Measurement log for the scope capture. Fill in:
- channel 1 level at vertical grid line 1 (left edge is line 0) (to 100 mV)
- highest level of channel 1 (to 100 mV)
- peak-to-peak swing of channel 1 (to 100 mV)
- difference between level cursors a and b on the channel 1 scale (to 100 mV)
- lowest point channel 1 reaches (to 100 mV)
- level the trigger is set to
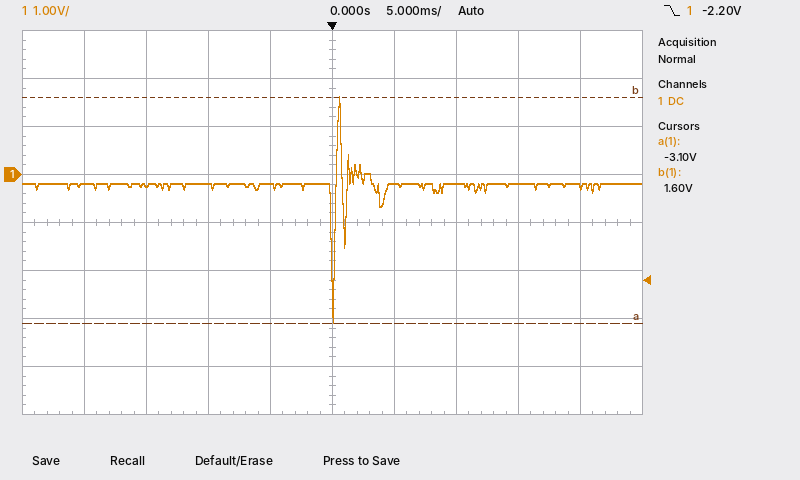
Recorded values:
-200 mV
1.6 V
4.7 V
4.7 V
-3.1 V
-2.20 V
